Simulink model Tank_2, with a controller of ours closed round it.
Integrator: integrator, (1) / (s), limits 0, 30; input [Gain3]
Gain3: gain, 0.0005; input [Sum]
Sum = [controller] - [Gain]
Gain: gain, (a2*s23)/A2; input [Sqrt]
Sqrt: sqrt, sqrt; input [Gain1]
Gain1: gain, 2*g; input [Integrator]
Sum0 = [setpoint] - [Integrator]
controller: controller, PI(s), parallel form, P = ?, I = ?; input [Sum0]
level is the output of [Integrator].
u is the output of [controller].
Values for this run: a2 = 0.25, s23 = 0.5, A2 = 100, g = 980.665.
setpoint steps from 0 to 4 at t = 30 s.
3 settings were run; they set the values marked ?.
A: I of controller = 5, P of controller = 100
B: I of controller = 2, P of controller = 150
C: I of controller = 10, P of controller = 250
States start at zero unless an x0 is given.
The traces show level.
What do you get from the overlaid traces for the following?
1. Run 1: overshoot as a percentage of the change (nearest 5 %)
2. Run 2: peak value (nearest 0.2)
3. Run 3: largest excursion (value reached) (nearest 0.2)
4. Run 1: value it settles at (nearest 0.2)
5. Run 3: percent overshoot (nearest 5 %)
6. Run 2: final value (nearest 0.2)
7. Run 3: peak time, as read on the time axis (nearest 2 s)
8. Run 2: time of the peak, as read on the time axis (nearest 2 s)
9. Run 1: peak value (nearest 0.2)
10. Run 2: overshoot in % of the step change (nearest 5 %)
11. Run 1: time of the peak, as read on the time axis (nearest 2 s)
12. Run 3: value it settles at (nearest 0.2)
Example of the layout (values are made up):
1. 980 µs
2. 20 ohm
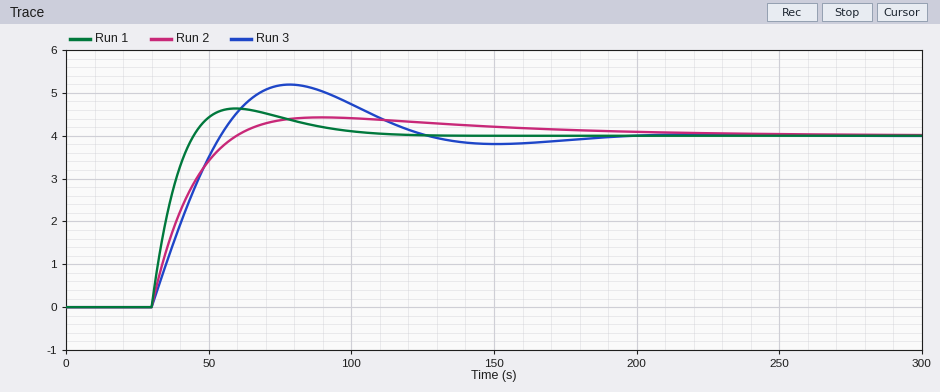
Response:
1. 15 %
2. 4.4
3. 5.2
4. 4.0
5. 30 %
6. 4.0
7. 78 s
8. 90 s
9. 4.6
10. 10 %
11. 60 s
12. 4.0
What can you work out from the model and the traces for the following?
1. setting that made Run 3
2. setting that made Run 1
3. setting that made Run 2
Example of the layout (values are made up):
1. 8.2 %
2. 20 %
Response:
1. A
2. C
3. B
